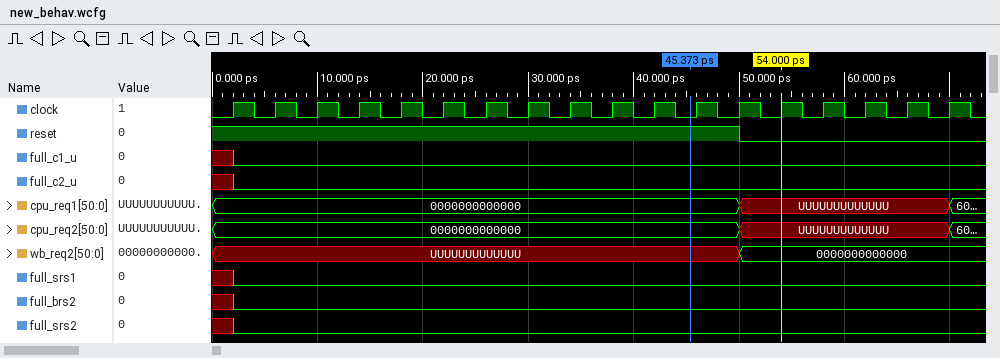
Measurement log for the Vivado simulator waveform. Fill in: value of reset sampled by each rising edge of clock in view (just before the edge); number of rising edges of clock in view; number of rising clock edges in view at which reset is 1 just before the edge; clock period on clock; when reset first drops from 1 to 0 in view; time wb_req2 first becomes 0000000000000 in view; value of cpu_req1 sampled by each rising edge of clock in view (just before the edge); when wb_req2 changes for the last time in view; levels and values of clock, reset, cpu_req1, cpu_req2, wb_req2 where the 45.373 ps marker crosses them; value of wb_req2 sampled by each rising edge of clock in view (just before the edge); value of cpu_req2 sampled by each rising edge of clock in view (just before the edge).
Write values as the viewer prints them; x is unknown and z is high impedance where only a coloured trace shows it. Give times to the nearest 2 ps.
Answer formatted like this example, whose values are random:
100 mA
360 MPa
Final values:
1 1 1 1 1 1 1 1 1 1 1 1 1 0 0 0 0 0
18
13
4 ps
50 ps
50 ps
0000000000000, 0000000000000, 0000000000000, 0000000000000, 0000000000000, 0000000000000, 0000000000000, 0000000000000, 0000000000000, 0000000000000, 0000000000000, 0000000000000, 0000000000000, UUUUUUUUUUUUU, UUUUUUUUUUUUU, UUUUUUUUUUUUU, UUUUUUUUUUUUU, UUUUUUUUUUUUU
50 ps
clock=0, reset=1, cpu_req1=0000000000000, cpu_req2=0000000000000, wb_req2=UUUUUUUUUUUUU
UUUUUUUUUUUUU, UUUUUUUUUUUUU, UUUUUUUUUUUUU, UUUUUUUUUUUUU, UUUUUUUUUUUUU, UUUUUUUUUUUUU, UUUUUUUUUUUUU, UUUUUUUUUUUUU, UUUUUUUUUUUUU, UUUUUUUUUUUUU, UUUUUUUUUUUUU, UUUUUUUUUUUUU, UUUUUUUUUUUUU, 0000000000000, 0000000000000, 0000000000000, 0000000000000, 0000000000000
0000000000000, 0000000000000, 0000000000000, 0000000000000, 0000000000000, 0000000000000, 0000000000000, 0000000000000, 0000000000000, 0000000000000, 0000000000000, 0000000000000, 0000000000000, UUUUUUUUUUUUU, UUUUUUUUUUUUU, UUUUUUUUUUUUU, UUUUUUUUUUUUU, UUUUUUUUUUUUU
